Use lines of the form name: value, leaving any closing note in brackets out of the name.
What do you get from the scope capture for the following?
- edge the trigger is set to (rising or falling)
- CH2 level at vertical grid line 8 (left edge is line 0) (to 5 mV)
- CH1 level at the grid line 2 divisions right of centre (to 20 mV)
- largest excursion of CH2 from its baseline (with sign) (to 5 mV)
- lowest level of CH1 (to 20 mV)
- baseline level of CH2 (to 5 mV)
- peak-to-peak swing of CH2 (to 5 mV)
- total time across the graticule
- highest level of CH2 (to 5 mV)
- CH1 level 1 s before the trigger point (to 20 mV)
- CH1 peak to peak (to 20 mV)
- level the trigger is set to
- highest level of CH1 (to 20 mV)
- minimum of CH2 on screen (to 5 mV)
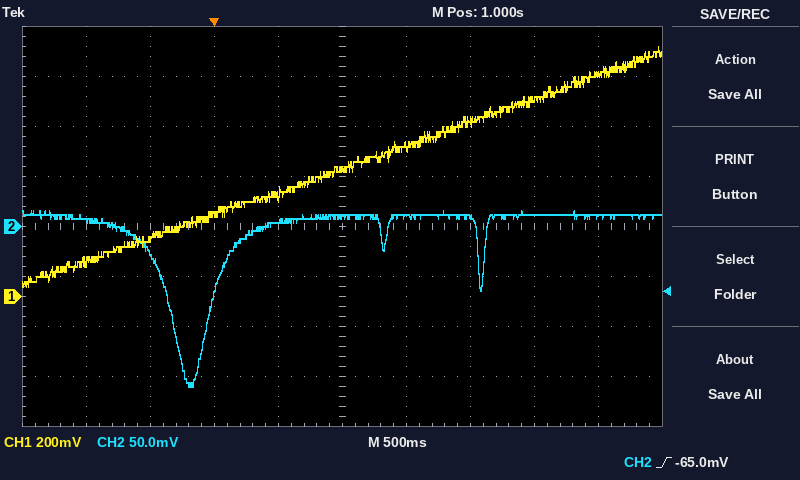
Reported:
edge the trigger is set to: rising
CH2 level at vertical grid line 8 (left edge is line 0): 10 mV
CH1 level at the grid line 2 divisions right of centre: 700 mV
largest excursion of CH2 from its baseline (with sign): -170 mV
lowest level of CH1: 40 mV
baseline level of CH2: 10 mV
peak-to-peak swing of CH2: 175 mV
total time across the graticule: 5 s
highest level of CH2: 15 mV
CH1 level 1 s before the trigger point: 140 mV
CH1 peak to peak: 960 mV
level the trigger is set to: -65.0 mV
highest level of CH1: 1.00 V
minimum of CH2 on screen: -160 mV
